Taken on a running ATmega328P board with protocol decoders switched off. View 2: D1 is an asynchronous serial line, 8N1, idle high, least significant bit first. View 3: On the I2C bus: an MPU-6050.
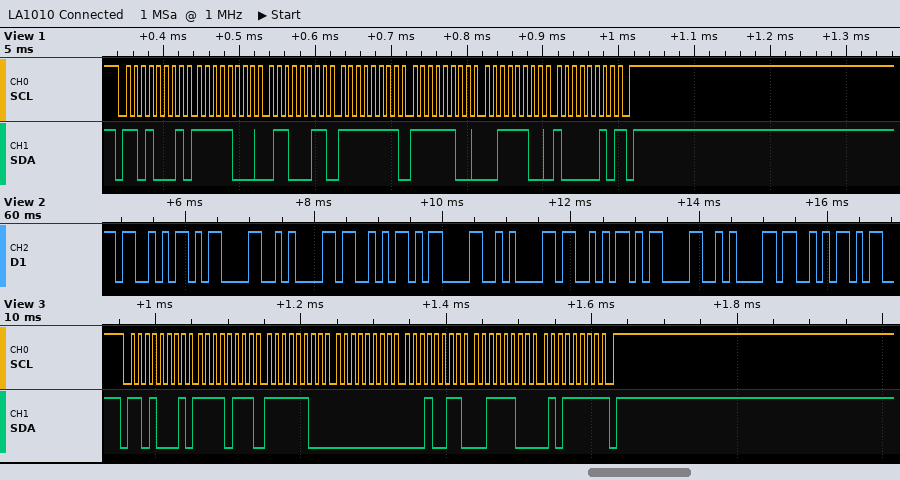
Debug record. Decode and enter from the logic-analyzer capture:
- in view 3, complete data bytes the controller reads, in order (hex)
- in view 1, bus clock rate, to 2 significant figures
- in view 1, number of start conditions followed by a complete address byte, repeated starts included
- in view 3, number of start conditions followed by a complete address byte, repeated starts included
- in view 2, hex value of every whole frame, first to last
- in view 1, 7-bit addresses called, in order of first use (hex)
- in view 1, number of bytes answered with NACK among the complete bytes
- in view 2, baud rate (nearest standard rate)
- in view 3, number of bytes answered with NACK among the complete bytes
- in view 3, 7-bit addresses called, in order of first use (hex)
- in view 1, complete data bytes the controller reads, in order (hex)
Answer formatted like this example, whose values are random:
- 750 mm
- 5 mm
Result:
- F7 FC 00 13 3C 5F
- 100 kHz
- 1
- 1
- 53 0D 0A 53 0D 0A 53 0D 0A 53
- 0x68
- 1
- 9600 baud
- 1
- 0x68
- F8 63 FF FC 3C 82
